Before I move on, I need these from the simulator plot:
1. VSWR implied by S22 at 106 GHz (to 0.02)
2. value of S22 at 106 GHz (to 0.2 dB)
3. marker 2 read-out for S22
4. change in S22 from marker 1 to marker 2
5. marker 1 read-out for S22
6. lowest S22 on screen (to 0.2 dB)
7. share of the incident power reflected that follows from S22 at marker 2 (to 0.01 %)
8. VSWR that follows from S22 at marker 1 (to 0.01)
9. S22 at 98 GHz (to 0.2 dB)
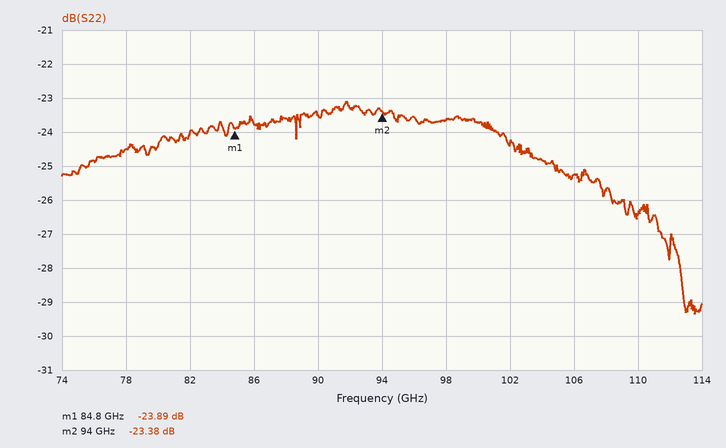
1.12
-25.2 dB
-23.38 dB
0.51 dB
-23.89 dB
-29.4 dB
0.46 %
1.14
-23.6 dB
